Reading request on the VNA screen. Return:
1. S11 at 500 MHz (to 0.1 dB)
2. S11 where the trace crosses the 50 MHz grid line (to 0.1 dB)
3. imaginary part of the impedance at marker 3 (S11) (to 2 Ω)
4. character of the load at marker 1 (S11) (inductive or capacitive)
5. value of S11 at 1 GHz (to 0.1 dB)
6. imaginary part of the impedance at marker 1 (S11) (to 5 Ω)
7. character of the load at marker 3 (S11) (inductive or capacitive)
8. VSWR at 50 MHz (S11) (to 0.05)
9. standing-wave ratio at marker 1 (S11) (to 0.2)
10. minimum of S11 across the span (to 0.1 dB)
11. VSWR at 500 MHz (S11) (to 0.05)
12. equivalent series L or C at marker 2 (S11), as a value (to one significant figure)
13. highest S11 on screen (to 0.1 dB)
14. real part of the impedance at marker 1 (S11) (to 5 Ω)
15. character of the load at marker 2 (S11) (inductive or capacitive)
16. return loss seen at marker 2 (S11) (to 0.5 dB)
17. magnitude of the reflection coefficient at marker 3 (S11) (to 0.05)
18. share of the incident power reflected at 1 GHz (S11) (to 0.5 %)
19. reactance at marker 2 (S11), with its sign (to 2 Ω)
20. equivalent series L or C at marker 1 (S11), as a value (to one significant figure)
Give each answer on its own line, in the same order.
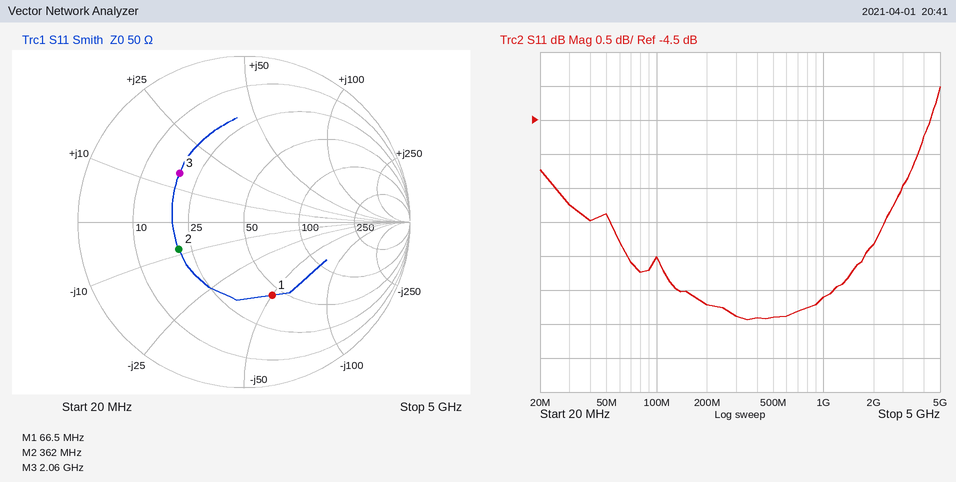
-7.4 dB
-5.9 dB
+14 Ω
capacitive
-7.1 dB
-50 Ω
inductive
3.05
2.8
-7.4 dB
2.50
50 pF
-4.0 dB
45 Ω
capacitive
7.5 dB
0.50
19.5 %
-8 Ω
50 pF
